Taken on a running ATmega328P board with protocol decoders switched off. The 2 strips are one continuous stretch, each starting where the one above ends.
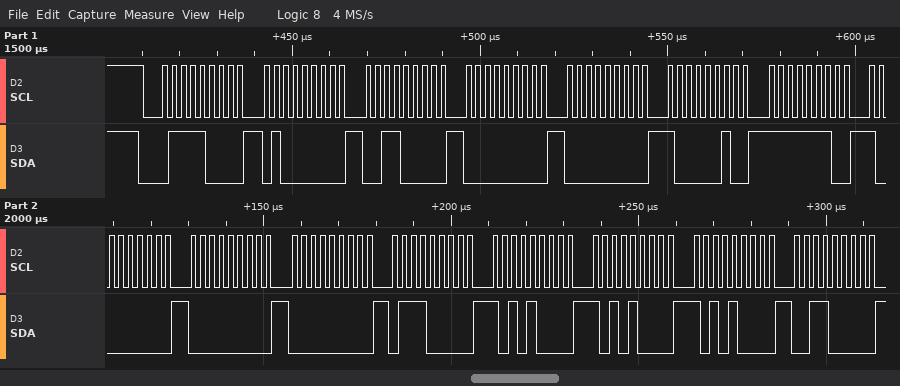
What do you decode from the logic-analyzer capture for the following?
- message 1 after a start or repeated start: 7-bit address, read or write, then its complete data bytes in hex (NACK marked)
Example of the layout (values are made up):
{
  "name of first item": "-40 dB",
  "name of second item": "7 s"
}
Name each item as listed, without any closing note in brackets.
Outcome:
{
  "message 1 after a start or repeated start: 7-bit address, read or write, then its complete data bytes in hex": "0x3C write: 40 30 00 00 82 FE 80 00 00 70 A8 A8 A8 30"
}
